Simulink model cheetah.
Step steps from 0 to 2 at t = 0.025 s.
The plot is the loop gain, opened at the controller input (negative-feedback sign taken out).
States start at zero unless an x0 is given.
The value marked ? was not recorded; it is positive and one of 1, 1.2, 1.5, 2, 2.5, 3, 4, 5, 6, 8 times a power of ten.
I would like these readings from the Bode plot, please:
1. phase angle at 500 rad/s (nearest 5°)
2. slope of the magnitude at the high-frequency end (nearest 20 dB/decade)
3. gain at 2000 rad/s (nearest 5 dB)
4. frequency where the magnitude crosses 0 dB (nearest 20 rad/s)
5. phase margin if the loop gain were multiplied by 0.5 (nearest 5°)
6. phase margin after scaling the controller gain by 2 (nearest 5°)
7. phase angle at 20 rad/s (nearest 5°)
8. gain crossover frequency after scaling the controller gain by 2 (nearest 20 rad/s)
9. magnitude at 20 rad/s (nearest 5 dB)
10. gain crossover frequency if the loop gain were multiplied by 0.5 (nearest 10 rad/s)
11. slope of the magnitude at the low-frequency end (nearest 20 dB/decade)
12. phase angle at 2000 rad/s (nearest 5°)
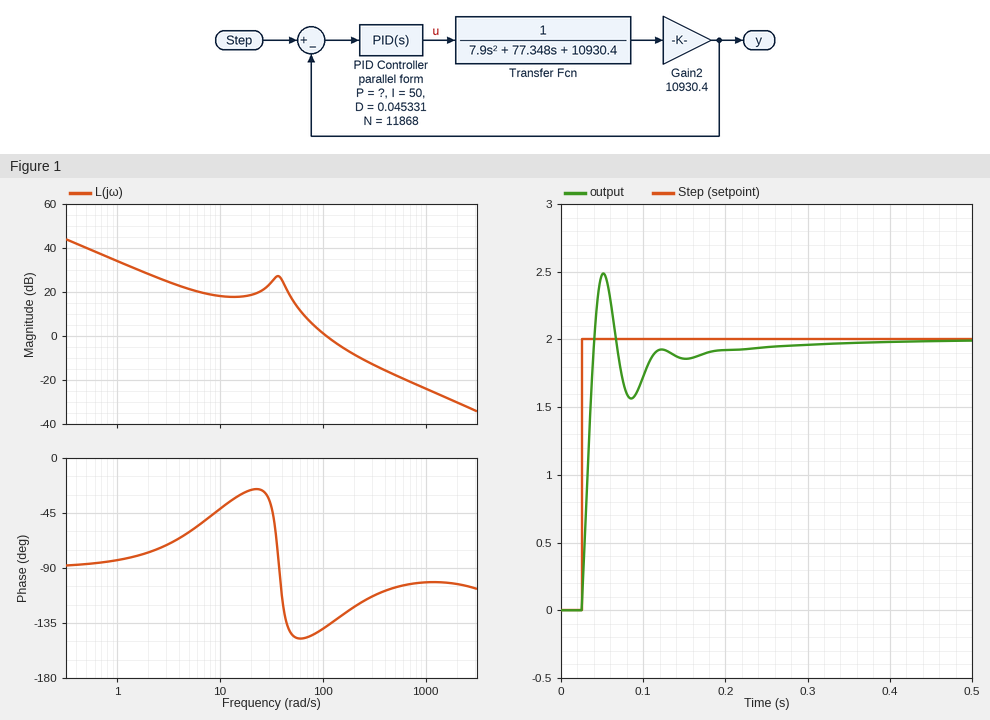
-105°
-20 dB/decade
-30 dB
100 rad/s
35°
55°
-25°
160 rad/s
20 dB
80 rad/s
-20 dB/decade
-105°
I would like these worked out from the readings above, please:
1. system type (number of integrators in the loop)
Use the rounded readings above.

1
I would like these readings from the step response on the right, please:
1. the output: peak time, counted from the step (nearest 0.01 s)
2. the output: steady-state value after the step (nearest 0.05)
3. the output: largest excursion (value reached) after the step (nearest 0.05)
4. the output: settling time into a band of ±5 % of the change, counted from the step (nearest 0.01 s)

0.03 s
2.00
2.50
0.15 s
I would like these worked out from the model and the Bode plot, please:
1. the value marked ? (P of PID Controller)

6
